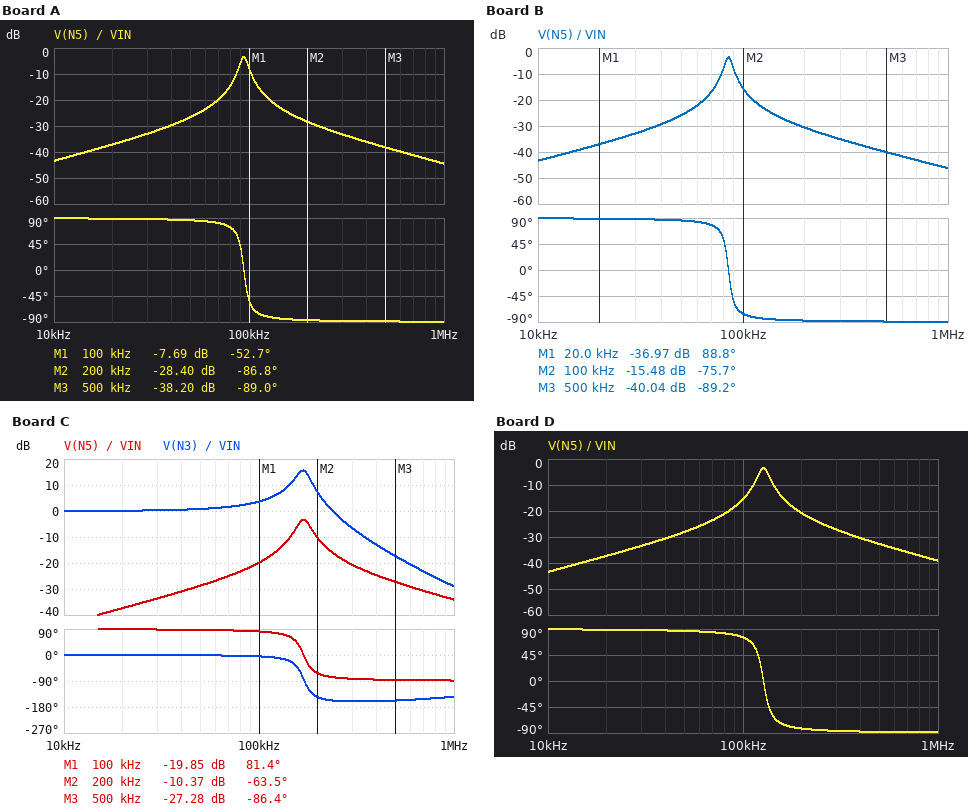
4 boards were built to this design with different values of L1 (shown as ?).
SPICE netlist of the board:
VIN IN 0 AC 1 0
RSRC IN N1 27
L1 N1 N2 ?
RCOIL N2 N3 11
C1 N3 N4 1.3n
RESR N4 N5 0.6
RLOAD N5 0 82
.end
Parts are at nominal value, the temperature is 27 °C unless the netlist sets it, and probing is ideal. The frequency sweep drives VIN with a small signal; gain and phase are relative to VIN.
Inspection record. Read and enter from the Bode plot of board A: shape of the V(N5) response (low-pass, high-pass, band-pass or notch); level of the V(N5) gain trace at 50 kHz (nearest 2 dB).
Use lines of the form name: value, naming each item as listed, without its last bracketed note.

shape of the V(N5) response: band-pass
level of the V(N5) gain trace at 50 kHz: -26 dB
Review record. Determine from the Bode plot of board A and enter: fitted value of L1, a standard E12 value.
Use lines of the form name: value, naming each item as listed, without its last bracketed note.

fitted value of L1, a standard E12 value: 2.2 mH
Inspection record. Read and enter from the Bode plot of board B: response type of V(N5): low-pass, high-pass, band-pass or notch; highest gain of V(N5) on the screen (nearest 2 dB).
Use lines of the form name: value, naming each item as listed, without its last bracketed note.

response type of V(N5): low-pass, high-pass, band-pass or notch: band-pass
highest gain of V(N5) on the screen: -4 dB
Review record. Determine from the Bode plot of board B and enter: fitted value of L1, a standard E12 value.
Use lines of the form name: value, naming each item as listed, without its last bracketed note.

fitted value of L1, a standard E12 value: 2.7 mH
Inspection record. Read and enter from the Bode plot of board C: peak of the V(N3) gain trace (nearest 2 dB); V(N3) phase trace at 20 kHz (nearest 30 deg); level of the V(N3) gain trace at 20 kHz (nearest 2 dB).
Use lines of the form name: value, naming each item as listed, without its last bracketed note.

peak of the V(N3) gain trace: 16 dB
V(N3) phase trace at 20 kHz: 0 deg
level of the V(N3) gain trace at 20 kHz: 0 dB
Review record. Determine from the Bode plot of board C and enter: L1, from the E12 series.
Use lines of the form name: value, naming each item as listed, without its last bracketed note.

L1, from the E12 series: 680 µH
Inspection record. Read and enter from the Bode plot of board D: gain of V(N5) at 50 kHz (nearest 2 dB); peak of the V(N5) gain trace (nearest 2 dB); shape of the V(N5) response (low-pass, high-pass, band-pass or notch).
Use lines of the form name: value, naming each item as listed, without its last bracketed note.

gain of V(N5) at 50 kHz: -28 dB
peak of the V(N5) gain trace: -4 dB
shape of the V(N5) response: band-pass
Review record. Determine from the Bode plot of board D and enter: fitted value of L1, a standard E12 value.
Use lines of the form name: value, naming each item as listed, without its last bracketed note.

fitted value of L1, a standard E12 value: 1.2 mH
